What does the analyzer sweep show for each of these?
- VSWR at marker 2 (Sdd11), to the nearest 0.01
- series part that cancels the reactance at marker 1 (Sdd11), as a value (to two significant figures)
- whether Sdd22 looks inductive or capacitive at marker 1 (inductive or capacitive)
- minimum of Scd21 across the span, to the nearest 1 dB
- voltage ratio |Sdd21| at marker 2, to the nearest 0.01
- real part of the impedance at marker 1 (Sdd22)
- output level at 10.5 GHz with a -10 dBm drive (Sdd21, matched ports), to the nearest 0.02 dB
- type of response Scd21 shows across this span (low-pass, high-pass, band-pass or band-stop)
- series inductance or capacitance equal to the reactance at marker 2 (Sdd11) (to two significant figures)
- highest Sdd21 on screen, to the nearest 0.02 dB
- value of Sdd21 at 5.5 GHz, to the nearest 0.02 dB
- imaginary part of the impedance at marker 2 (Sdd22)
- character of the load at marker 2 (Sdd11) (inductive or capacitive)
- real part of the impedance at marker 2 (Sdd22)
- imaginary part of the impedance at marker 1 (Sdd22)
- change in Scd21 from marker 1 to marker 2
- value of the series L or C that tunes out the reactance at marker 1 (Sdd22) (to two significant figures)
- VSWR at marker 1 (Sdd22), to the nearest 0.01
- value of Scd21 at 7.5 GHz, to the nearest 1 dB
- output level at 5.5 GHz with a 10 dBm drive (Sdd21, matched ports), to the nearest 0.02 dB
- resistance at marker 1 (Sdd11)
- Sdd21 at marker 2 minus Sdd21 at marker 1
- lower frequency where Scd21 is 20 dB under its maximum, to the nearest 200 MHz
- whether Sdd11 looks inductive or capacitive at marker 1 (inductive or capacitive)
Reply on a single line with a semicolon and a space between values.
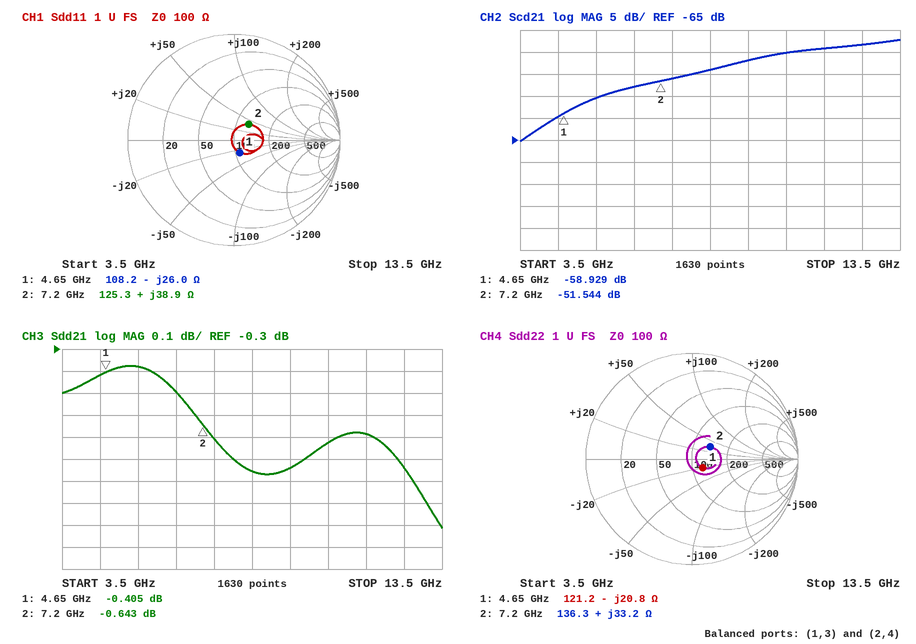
1.51; 890 pH; capacitive; -65 dB; 0.93; 121.2 Ω; -10.72 dBm; high-pass; 860 pH; -0.38 dB; -0.38 dB; +33.2 Ω; inductive; 136.3 Ω; -20.8 Ω; 7.385 dB; 710 pH; 1.31; -51 dB; 9.62 dBm; 108.2 Ω; -0.238 dB; 4.0 GHz; capacitive
